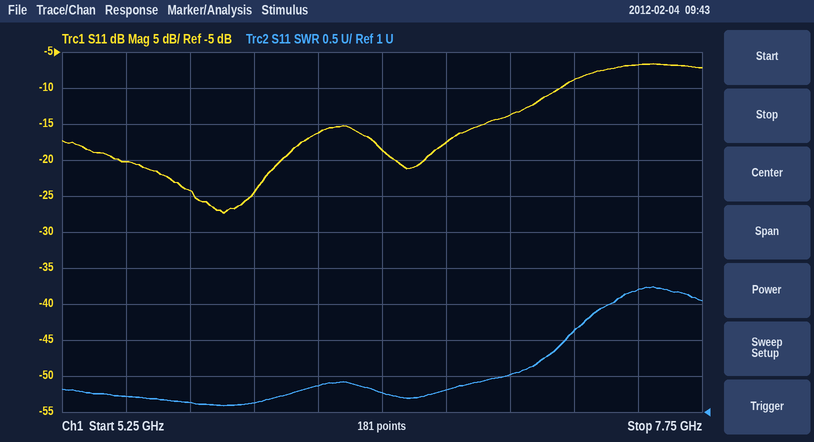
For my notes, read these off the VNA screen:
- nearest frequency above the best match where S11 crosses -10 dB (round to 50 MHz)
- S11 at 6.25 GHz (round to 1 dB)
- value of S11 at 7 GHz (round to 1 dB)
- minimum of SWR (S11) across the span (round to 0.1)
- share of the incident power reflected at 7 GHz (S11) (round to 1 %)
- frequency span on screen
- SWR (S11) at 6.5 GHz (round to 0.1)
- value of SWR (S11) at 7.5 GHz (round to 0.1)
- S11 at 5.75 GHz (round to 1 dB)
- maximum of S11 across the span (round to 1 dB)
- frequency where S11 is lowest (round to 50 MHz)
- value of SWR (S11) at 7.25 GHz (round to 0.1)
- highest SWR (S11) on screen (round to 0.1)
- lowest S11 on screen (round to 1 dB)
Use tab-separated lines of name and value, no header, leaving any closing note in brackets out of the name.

nearest frequency above the best match where S11 crosses -10 dB	7.20 GHz
S11 at 6.25 GHz	-16 dB
value of S11 at 7 GHz	-14 dB
minimum of SWR (S11) across the span	1.1
share of the incident power reflected at 7 GHz (S11)	4 %
frequency span on screen	2.5 GHz
SWR (S11) at 6.5 GHz	1.3
value of SWR (S11) at 7.5 GHz	2.7
S11 at 5.75 GHz	-24 dB
maximum of S11 across the span	-7 dB
frequency where S11 is lowest	5.90 GHz
value of SWR (S11) at 7.25 GHz	2.1
highest SWR (S11) on screen	2.7
lowest S11 on screen	-27 dB
